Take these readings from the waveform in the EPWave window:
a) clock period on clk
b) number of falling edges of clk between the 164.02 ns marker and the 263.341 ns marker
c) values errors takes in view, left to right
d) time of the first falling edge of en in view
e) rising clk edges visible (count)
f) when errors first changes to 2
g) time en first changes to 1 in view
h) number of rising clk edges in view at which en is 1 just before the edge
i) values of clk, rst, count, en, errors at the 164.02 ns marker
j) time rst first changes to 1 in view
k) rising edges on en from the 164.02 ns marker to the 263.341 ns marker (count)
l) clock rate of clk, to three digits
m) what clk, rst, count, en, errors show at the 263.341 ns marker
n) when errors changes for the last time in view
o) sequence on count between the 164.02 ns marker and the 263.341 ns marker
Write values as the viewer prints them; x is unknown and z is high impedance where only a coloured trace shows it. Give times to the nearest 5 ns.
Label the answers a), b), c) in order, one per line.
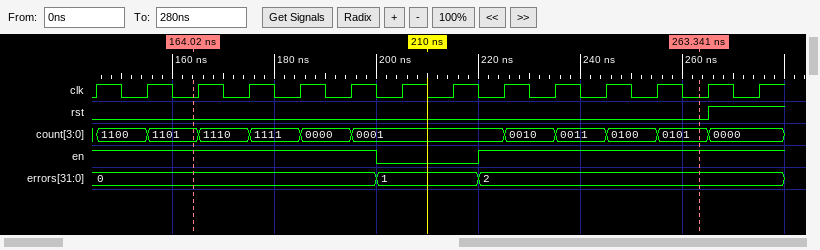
a) 10 ns
b) 10
c) 0, 1, 2
d) 200 ns
e) 14
f) 220 ns
g) 220 ns
h) 12
i) clk=0, rst=0, count=1101, en=1, errors=0
j) 265 ns
k) 1
l) 100 MHz
m) clk=0, rst=0, count=0101, en=1, errors=2
n) 220 ns
o) 1101, 1110, 1111, 0000, 0001, 0010, 0011, 0100, 0101
